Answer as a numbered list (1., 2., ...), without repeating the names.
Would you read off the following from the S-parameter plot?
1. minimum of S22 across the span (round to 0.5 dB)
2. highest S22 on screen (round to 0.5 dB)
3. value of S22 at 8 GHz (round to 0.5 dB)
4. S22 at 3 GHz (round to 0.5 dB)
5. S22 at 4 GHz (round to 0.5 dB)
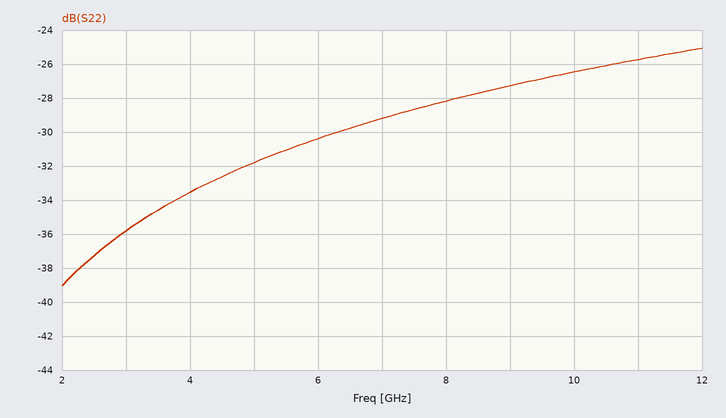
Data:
1. -39.0 dB
2. -25.0 dB
3. -28.0 dB
4. -36.0 dB
5. -33.5 dB
